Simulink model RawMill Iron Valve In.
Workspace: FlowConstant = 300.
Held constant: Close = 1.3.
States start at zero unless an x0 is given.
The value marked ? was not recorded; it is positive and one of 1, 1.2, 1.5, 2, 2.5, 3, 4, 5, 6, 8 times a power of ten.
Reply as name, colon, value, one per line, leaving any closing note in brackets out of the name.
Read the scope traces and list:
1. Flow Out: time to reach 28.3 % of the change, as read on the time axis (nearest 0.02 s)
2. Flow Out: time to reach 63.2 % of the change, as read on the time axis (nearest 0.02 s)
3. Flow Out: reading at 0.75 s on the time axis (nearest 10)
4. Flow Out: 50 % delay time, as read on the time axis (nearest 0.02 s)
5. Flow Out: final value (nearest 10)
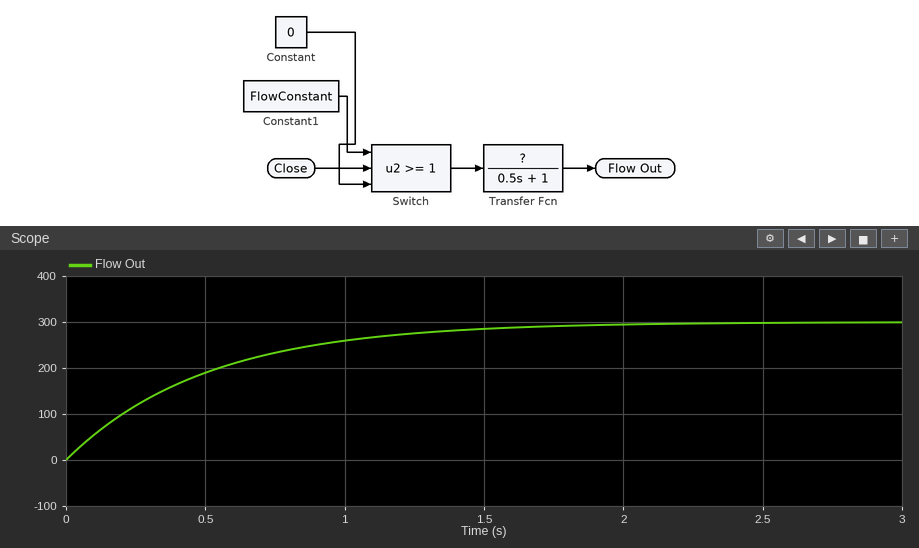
Flow Out: time to reach 28.3 % of the change, as read on the time axis: 0.16 s
Flow Out: time to reach 63.2 % of the change, as read on the time axis: 0.50 s
Flow Out: reading at 0.75 s on the time axis: 230
Flow Out: 50 % delay time, as read on the time axis: 0.34 s
Flow Out: final value: 300
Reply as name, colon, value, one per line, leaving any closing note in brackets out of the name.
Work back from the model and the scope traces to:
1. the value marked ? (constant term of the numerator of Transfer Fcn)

the value marked ?: 1
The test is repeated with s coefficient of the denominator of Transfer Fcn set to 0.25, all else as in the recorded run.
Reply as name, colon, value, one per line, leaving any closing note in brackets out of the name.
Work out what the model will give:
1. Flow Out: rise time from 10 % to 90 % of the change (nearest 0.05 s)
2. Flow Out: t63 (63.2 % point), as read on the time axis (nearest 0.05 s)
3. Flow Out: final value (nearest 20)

Flow Out: rise time from 10 % to 90 % of the change: 0.55 s
Flow Out: t63 (63.2 % point), as read on the time axis: 0.25 s
Flow Out: final value: 300
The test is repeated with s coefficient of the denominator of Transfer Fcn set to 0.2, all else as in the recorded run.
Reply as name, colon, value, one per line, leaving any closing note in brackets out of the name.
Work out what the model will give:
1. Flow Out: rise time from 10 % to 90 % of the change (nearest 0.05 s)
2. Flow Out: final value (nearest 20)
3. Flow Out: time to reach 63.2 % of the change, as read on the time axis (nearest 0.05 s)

Flow Out: rise time from 10 % to 90 % of the change: 0.45 s
Flow Out: final value: 300
Flow Out: time to reach 63.2 % of the change, as read on the time axis: 0.20 s
